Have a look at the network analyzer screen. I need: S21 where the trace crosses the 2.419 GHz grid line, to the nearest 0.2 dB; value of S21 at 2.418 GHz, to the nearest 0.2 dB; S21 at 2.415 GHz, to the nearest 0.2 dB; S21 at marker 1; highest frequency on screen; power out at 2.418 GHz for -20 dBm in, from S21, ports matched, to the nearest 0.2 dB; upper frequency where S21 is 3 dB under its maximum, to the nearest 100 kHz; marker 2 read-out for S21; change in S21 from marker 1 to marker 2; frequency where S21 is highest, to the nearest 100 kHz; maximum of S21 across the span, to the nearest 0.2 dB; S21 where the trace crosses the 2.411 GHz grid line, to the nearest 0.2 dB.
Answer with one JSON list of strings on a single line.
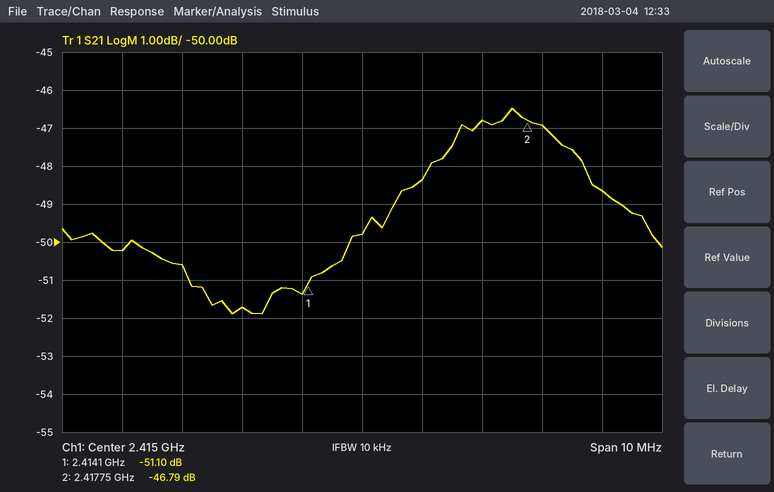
["-48.6 dB", "-47.0 dB", "-49.8 dB", "-51.10 dB", "2.42 GHz", "-67.0 dBm", "2.4197 GHz", "-46.79 dB", "4.31 dB", "2.4175 GHz", "-46.4 dB", "-50.2 dB"]
